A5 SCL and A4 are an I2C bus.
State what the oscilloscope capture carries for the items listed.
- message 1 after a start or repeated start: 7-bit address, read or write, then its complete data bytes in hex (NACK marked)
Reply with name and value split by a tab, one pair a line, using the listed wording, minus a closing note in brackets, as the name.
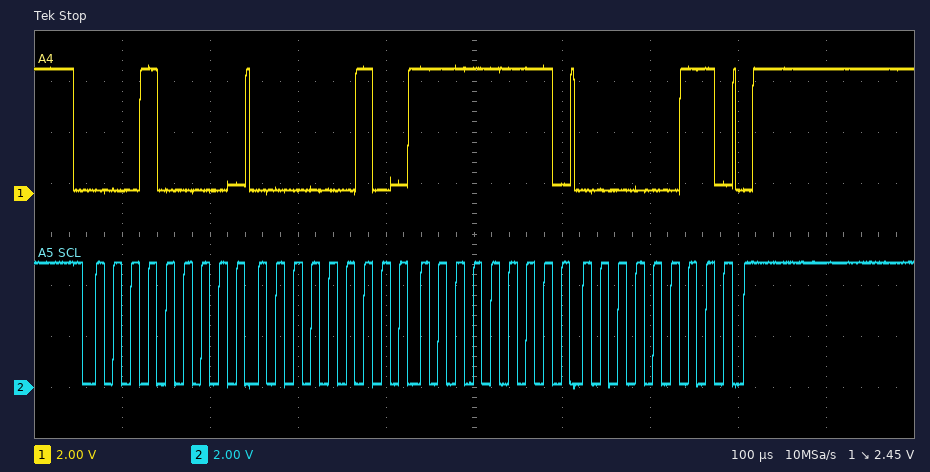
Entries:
message 1 after a start or repeated start: 7-bit address, read or write, then its complete data bytes in hex	0x08 write: 02 FF 03
